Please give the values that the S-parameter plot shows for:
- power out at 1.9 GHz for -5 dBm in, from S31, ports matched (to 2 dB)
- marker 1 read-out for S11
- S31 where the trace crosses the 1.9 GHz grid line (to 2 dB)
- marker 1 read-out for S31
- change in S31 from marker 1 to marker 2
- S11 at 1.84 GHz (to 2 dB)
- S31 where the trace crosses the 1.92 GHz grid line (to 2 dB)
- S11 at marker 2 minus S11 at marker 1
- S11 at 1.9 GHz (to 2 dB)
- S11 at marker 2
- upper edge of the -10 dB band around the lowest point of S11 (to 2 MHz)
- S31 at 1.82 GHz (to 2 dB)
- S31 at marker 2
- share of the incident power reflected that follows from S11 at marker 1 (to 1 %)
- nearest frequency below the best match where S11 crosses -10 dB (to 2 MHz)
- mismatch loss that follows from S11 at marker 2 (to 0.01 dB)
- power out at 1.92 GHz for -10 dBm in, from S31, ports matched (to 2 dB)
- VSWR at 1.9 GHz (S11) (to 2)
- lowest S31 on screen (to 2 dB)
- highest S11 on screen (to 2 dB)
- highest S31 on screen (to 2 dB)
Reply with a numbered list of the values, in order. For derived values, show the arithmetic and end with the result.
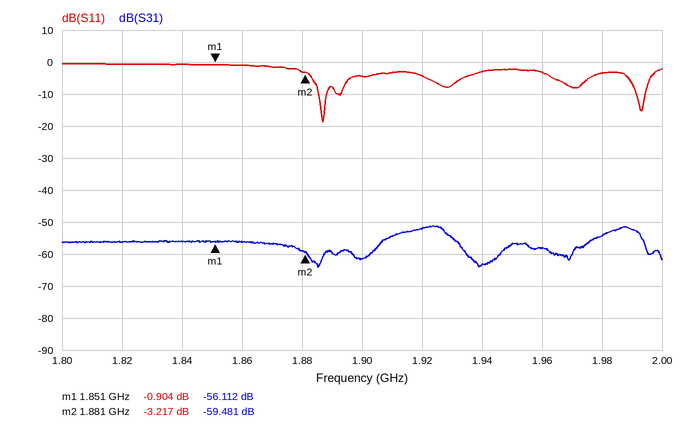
1. -5 dBm + (-62 dB) = -66 dBm
2. -0.904 dB
3. -62 dB
4. -56.112 dB
5. -59.481 − (-56.112) = -3.369 dB
6. 0 dB
7. -52 dB
8. -3.217 − (-0.904) = -2.313 dB
9. -4 dB
10. -3.217 dB
11. 1.888 GHz
12. -56 dB
13. -59.481 dB
14. 10^(-0.904/10) ≈ 81 %
15. 1.886 GHz
16. −10 log10(1 − 10^(-3.217/10)) ≈ 2.81 dB
17. -10 dBm + (-52 dB) = -62 dBm
18. |Γ| = 10^(-4/20) = 0.6310; VSWR = (1 + 0.6310)/(1 − 0.6310) ≈ 4
19. -64 dB
20. 0 dB
21. -52 dB
